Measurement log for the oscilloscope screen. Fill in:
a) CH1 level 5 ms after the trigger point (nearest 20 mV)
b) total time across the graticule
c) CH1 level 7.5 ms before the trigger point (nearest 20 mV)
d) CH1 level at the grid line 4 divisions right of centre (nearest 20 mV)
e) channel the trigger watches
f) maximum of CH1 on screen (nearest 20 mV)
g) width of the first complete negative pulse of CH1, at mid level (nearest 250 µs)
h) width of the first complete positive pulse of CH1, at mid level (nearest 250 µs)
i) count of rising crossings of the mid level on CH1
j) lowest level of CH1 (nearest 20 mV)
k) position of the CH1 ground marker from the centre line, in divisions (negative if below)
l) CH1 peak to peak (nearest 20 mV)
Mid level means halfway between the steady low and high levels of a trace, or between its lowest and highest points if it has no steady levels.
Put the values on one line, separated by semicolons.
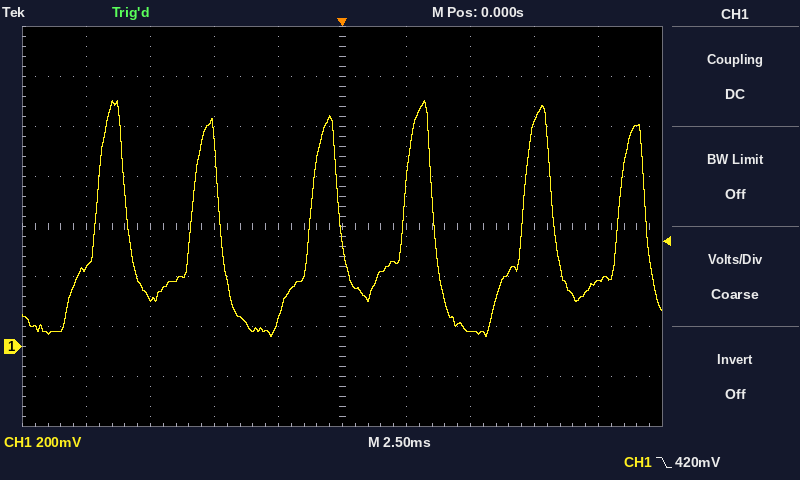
60 mV; 25 ms; 200 mV; 260 mV; CH1; 980 mV; 2.50 ms; 1.25 ms; 6; 40 mV; -2.4 div; 940 mV
